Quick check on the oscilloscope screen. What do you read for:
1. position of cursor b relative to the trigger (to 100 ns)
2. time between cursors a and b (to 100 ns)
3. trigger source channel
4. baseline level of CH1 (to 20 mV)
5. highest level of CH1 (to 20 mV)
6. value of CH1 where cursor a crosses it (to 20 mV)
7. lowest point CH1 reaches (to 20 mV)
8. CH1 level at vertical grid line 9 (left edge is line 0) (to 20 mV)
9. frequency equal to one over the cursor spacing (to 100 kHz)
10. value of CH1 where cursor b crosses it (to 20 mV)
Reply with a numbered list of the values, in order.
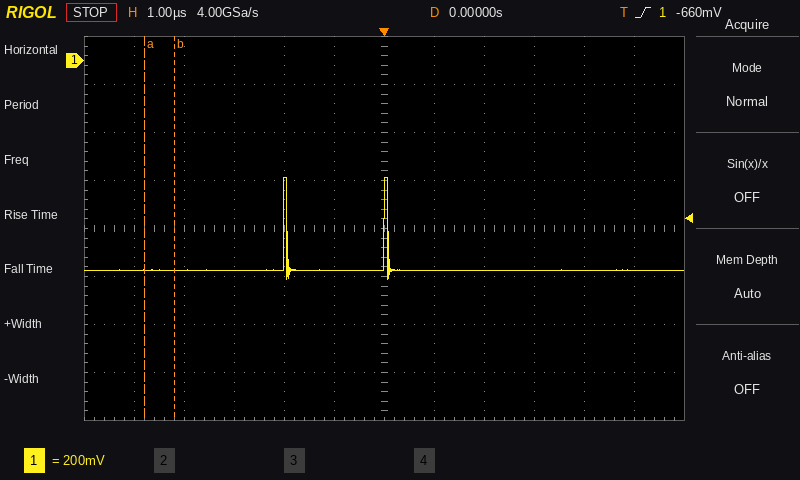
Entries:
1. -4.2 µs
2. 600 ns
3. CH1
4. -880 mV
5. -480 mV
6. -880 mV
7. -920 mV
8. -880 mV
9. 1.7 MHz
10. -880 mV
